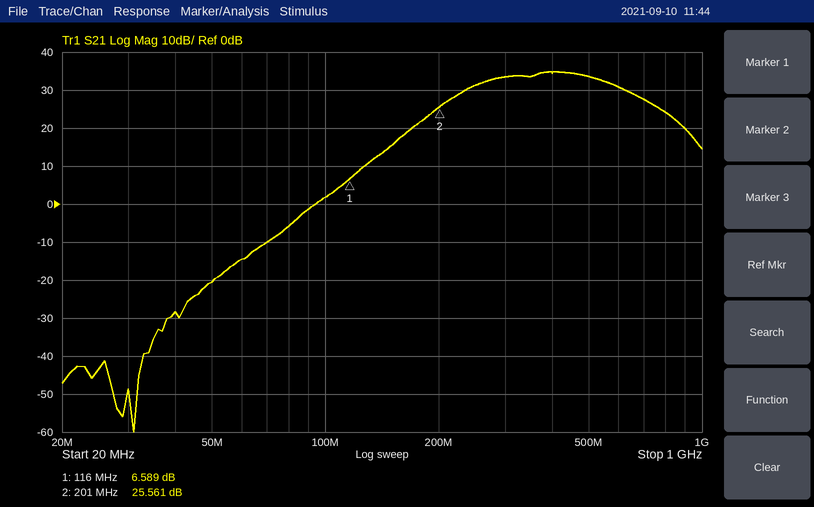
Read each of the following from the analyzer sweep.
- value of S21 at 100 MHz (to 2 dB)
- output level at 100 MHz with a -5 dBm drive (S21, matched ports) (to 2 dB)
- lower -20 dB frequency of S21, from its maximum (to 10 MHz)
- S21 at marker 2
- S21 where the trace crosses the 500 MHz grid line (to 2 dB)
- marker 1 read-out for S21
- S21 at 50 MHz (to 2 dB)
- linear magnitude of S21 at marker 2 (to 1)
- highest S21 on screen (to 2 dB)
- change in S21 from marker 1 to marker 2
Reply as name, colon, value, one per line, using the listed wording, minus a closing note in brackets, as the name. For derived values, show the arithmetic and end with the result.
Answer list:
value of S21 at 100 MHz: 2 dB
output level at 100 MHz with a -5 dBm drive (S21, matched ports): -5 dBm + (2 dB) = -4 dBm
lower -20 dB frequency of S21, from its maximum: 150 MHz
S21 at marker 2: 25.561 dB
S21 where the trace crosses the 500 MHz grid line: 34 dB
marker 1 read-out for S21: 6.589 dB
S21 at 50 MHz: -20 dB
linear magnitude of S21 at marker 2: 10^(25.561/20) ≈ 19
highest S21 on screen: 34 dB
change in S21 from marker 1 to marker 2: 25.561 − (6.589) = 18.972 dB
